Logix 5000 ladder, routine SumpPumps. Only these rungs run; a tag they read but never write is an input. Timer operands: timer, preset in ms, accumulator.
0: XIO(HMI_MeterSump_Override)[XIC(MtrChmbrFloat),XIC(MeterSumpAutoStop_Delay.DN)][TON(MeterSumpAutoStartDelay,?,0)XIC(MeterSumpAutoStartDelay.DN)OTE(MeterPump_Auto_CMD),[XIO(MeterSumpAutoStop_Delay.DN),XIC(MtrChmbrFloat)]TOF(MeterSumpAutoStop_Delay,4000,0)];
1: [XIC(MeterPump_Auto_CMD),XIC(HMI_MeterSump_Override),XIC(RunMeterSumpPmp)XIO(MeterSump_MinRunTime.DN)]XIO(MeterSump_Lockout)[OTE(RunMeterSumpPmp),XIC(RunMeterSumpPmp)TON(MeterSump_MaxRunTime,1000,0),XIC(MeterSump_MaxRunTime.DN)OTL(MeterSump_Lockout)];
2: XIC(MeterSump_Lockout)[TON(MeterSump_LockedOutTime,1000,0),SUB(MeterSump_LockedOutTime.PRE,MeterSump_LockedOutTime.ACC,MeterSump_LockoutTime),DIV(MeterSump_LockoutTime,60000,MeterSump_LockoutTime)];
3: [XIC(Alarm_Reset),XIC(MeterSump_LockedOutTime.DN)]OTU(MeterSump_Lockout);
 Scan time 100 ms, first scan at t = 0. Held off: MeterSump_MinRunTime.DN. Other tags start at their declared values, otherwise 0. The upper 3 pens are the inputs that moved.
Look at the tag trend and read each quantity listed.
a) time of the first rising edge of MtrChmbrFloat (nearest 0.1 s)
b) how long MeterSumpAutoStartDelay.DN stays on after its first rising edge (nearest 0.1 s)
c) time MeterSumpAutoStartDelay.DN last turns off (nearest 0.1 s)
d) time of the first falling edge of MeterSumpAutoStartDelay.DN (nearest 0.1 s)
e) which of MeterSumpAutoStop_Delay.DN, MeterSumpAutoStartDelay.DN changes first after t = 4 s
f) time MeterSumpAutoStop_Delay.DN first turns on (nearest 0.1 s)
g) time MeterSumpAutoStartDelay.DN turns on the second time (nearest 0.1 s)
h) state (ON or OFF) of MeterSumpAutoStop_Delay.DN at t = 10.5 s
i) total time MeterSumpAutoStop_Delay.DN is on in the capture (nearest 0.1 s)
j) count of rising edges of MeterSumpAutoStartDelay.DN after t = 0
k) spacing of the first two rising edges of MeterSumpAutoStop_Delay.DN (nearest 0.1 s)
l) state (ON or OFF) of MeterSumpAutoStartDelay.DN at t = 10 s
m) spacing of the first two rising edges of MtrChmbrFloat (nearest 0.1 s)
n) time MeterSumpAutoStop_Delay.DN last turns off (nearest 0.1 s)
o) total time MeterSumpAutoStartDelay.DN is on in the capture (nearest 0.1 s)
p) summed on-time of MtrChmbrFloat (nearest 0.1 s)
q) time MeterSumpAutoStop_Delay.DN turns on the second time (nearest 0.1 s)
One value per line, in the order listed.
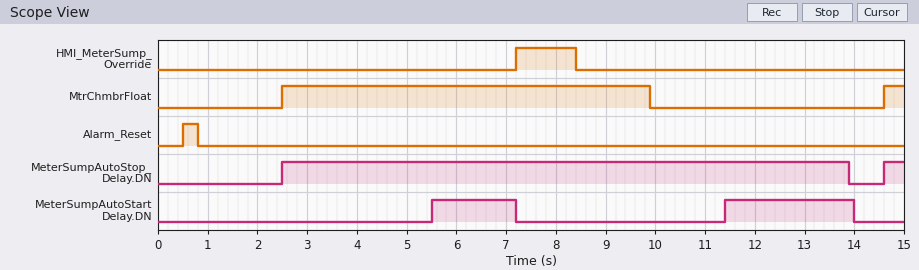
2.5 s
1.7 s
14.0 s
7.2 s
MeterSumpAutoStartDelay.DN
2.5 s
11.4 s
ON
11.8 s
2
12.1 s
OFF
12.1 s
13.9 s
4.3 s
7.8 s
14.6 s
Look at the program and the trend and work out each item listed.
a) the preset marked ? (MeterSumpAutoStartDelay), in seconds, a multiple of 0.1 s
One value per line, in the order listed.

3.0 s
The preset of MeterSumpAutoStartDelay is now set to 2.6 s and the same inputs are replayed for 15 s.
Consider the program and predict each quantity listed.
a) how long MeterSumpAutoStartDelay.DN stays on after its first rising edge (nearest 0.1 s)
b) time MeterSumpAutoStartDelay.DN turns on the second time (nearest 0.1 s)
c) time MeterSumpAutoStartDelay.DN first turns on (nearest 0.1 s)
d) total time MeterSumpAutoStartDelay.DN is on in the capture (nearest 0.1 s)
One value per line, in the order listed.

2.1 s
11.0 s
5.1 s
5.1 s
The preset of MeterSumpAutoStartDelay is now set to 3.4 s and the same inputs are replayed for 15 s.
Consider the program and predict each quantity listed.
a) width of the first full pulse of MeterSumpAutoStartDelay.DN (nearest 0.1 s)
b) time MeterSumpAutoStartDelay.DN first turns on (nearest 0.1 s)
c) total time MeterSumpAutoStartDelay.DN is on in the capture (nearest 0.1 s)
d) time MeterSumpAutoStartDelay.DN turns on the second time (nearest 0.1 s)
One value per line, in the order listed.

1.3 s
5.9 s
3.5 s
11.8 s
